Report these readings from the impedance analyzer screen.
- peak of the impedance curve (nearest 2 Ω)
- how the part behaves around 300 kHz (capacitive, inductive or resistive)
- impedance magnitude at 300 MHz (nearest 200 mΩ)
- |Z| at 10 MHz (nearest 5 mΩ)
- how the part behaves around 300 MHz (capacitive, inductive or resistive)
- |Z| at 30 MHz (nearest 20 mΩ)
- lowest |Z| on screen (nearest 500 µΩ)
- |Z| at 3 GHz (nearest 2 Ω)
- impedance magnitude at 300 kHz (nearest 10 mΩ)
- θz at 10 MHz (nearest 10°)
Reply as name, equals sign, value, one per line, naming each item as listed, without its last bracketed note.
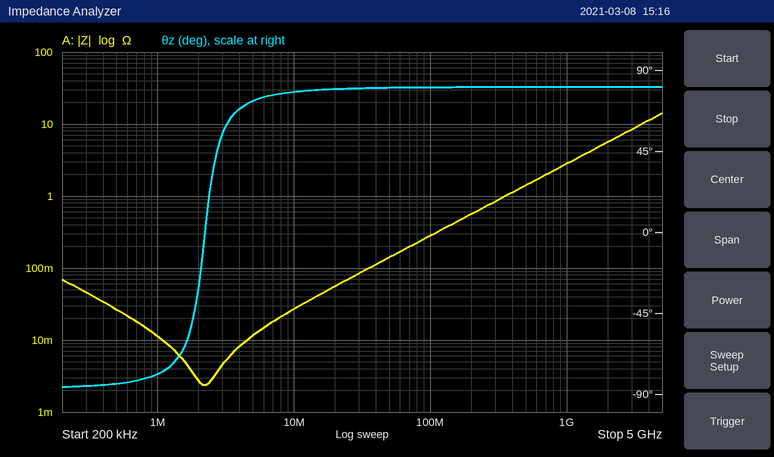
peak of the impedance curve = 14 Ω
how the part behaves around 300 kHz = capacitive
impedance magnitude at 300 MHz = 800 mΩ
|Z| at 10 MHz = 25 mΩ
how the part behaves around 300 MHz = inductive
|Z| at 30 MHz = 80 mΩ
lowest |Z| on screen = 2.5 mΩ
|Z| at 3 GHz = 8 Ω
impedance magnitude at 300 kHz = 50 mΩ
θz at 10 MHz = 80°
